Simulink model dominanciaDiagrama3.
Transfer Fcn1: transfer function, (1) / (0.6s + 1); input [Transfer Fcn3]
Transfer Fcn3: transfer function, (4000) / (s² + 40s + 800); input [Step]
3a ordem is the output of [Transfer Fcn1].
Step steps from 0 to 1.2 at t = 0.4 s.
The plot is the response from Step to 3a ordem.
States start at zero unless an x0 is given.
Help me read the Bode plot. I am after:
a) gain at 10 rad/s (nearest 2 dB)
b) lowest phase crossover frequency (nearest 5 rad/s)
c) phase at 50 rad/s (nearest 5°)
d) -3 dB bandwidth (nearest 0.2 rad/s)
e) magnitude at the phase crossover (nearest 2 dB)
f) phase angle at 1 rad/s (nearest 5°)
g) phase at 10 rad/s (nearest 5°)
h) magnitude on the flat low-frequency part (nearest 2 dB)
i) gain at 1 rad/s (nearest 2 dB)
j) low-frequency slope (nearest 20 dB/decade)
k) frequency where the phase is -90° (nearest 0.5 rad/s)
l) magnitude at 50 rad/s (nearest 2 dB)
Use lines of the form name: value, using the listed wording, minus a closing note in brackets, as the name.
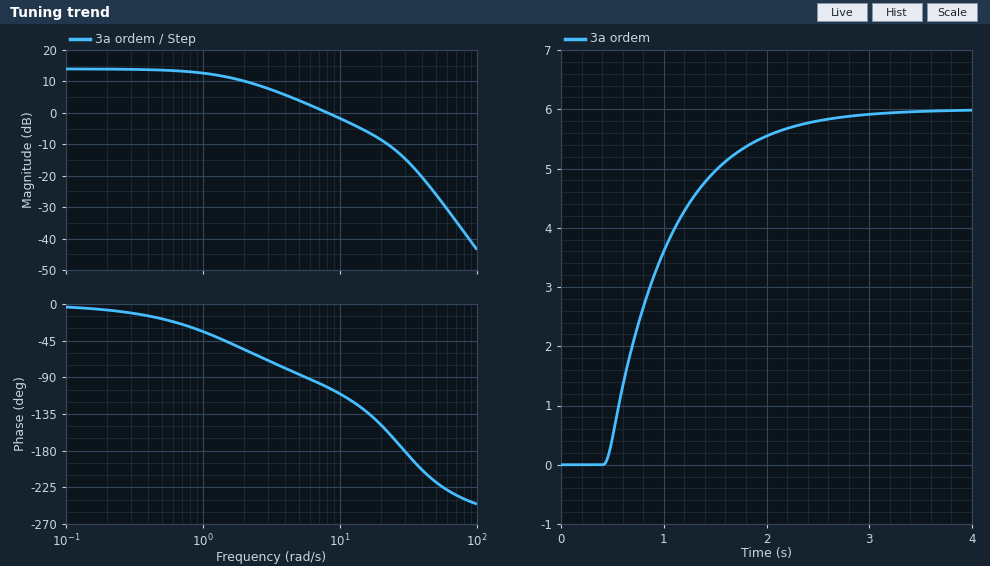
gain at 10 rad/s: -2 dB
lowest phase crossover frequency: 30 rad/s
phase at 50 rad/s: -220°
-3 dB bandwidth: 1.6 rad/s
magnitude at the phase crossover: -14 dB
phase angle at 1 rad/s: -35°
phase at 10 rad/s: -110°
magnitude on the flat low-frequency part: 14 dB
gain at 1 rad/s: 12 dB
low-frequency slope: 0 dB/decade
frequency where the phase is -90°: 5.5 rad/s
magnitude at 50 rad/s: -26 dB
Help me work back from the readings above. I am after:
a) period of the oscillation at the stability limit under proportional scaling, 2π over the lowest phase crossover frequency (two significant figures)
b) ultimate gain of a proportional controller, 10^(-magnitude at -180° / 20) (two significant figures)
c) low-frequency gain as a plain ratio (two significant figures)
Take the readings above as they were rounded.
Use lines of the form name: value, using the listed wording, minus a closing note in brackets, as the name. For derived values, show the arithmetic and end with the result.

period of the oscillation at the stability limit under proportional scaling, 2π over the lowest phase crossover frequency: 2π / 30 = 0.21 s
ultimate gain of a proportional controller, 10^(-magnitude at -180° / 20): 10^(14 / 20) = 5.0
low-frequency gain as a plain ratio: 10^(14 / 20) = 5.0
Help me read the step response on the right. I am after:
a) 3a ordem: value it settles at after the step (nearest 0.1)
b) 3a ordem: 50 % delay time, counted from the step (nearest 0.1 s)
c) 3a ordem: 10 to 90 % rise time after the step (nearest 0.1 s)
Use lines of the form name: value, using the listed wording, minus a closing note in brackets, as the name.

3a ordem: value it settles at after the step: 6.0
3a ordem: 50 % delay time, counted from the step: 0.5 s
3a ordem: 10 to 90 % rise time after the step: 1.3 s
